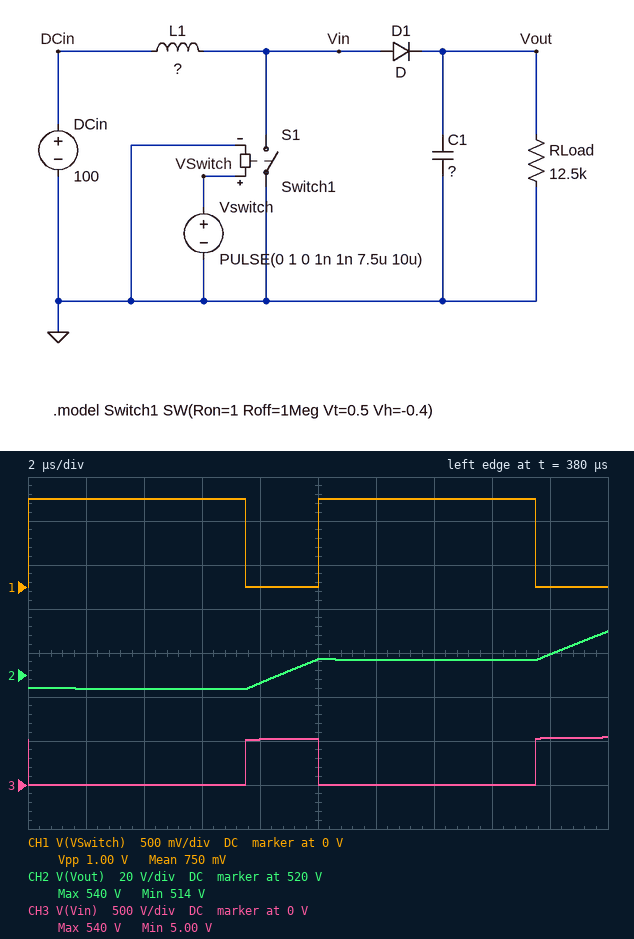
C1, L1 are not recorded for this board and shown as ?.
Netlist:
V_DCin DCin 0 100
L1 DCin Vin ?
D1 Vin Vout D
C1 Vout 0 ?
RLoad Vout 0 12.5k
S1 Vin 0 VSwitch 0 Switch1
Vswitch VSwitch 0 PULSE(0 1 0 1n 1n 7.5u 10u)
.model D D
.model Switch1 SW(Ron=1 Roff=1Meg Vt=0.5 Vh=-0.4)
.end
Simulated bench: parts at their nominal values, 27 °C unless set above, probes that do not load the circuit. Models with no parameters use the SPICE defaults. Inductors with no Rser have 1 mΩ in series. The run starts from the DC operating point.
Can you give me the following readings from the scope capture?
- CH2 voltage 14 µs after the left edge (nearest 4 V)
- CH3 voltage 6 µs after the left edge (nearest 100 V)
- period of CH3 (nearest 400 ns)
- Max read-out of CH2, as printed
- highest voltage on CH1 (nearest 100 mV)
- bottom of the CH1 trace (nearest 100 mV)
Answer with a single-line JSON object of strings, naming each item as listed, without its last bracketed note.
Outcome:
{"CH2 voltage 14 µs after the left edge": "528 V", "CH3 voltage 6 µs after the left edge": "0 V", "period of CH3": "10.0 µs", "Max read-out of CH2, as printed": "540 V", "highest voltage on CH1": "1.0 V", "bottom of the CH1 trace": "0 V"}
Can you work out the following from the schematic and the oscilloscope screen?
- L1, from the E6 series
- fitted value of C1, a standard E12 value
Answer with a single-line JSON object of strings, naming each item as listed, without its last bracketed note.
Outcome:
{"L1, from the E6 series": "3.3 mH", "fitted value of C1, a standard E12 value": "680 nF"}
